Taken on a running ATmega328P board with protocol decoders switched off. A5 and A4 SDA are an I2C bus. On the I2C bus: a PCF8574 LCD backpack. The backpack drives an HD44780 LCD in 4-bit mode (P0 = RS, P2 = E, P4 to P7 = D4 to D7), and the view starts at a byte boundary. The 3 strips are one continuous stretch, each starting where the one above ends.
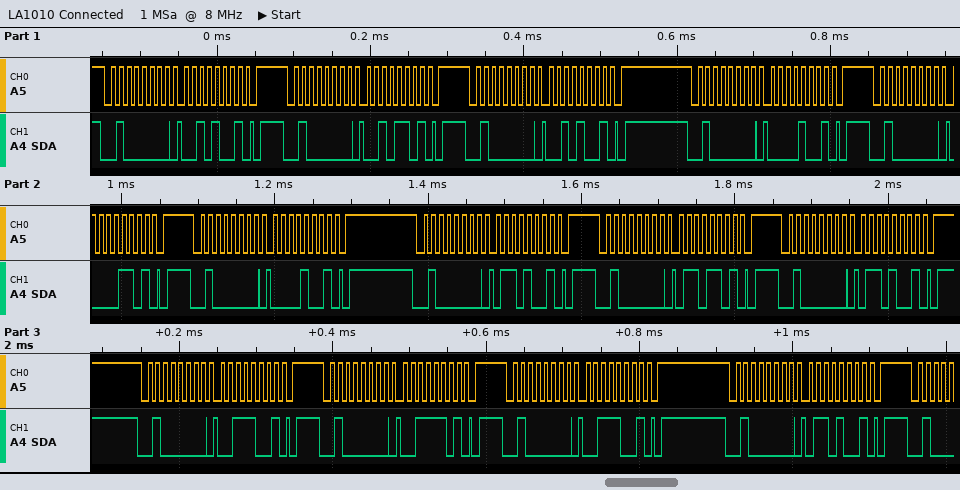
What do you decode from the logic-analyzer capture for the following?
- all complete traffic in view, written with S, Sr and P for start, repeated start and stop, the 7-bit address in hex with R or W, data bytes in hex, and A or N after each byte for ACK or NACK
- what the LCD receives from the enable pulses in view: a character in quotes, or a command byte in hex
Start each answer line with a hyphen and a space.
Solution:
- S 20W A 29 A P S 20W A 2D A P S 20W A 29 A P S 20W A 09 A P S 20W A 0D A P S 20W A 09 A P S 20W A 69 A P S 20W A 6D A P S 20W A 69 A P S 20W A 39 A P S 20W A 3D A P S 20W A 39 A P S 20W A 69 A P
- ' ' 'c'
